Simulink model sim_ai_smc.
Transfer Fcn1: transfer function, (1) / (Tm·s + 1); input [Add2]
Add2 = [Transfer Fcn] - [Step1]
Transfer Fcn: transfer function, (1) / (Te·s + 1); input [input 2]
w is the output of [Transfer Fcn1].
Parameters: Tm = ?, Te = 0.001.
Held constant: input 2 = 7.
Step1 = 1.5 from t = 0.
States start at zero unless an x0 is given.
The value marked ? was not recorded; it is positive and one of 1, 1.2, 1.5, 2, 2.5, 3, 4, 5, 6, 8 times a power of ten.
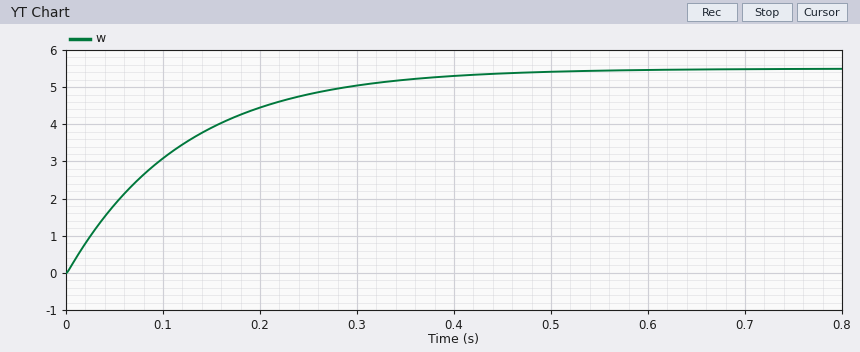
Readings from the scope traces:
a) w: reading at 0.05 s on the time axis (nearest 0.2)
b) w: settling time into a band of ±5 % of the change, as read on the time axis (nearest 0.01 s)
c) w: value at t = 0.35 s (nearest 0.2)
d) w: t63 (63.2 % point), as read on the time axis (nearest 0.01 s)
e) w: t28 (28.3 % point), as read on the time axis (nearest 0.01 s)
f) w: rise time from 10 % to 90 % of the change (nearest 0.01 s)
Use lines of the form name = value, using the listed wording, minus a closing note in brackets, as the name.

w: reading at 0.05 s on the time axis = 1.8
w: settling time into a band of ±5 % of the change, as read on the time axis = 0.36 s
w: value at t = 0.35 s = 5.2
w: t63 (63.2 % point), as read on the time axis = 0.12 s
w: t28 (28.3 % point), as read on the time axis = 0.04 s
w: rise time from 10 % to 90 % of the change = 0.26 s
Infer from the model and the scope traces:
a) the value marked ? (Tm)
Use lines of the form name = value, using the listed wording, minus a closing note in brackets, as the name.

the value marked ? = 0.12
